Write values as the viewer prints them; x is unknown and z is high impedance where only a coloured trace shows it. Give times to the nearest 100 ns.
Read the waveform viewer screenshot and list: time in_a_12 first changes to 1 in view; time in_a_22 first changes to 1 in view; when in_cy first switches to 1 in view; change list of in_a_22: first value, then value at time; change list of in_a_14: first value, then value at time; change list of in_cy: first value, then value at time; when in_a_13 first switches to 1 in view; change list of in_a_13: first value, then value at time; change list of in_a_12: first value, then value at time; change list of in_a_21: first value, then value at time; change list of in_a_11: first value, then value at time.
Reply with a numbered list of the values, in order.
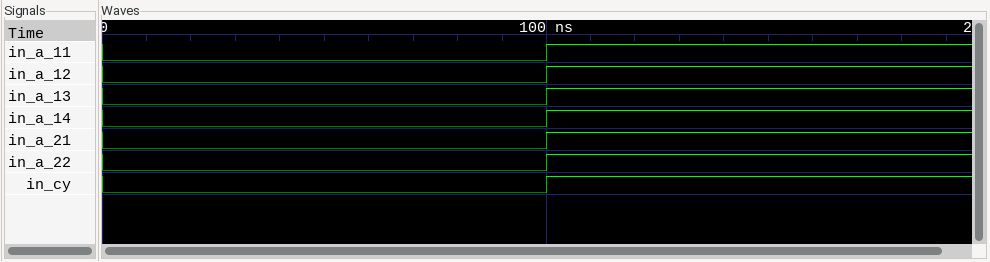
1. 100 ns
2. 100 ns
3. 100 ns
4. 0, 1 at 100 ns
5. 0, 1 at 100 ns
6. 0, 1 at 100 ns
7. 100 ns
8. 0, 1 at 100 ns
9. 0, 1 at 100 ns
10. 0, 1 at 100 ns
11. 0, 1 at 100 ns
